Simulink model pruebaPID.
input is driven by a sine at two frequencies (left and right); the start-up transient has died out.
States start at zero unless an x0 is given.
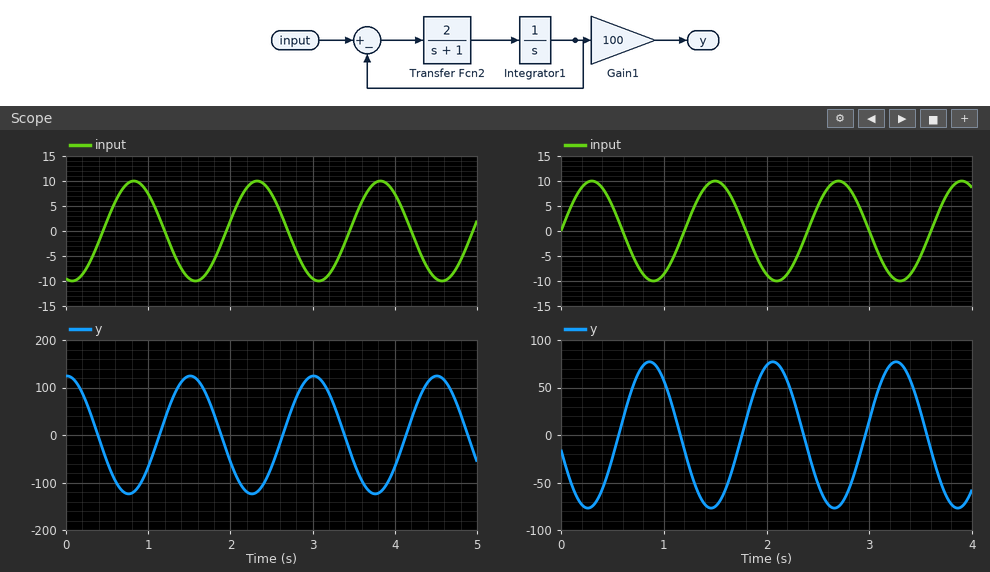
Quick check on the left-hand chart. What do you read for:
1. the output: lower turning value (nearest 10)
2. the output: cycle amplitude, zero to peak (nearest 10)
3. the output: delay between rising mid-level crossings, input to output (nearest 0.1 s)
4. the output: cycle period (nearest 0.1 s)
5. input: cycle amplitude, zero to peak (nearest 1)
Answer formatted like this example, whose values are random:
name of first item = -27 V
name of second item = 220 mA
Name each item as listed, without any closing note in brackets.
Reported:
the output: lower turning value = -120
the output: cycle amplitude, zero to peak = 120
the output: delay between rising mid-level crossings, input to output = 0.7 s
the output: cycle period = 1.5 s
input: cycle amplitude, zero to peak = 10
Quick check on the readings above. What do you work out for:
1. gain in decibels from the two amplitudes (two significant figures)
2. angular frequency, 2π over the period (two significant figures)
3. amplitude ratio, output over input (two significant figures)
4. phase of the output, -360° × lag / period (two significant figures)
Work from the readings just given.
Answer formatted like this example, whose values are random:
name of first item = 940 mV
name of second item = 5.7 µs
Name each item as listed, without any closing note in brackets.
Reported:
gain in decibels from the two amplitudes = 22 dB
angular frequency, 2π over the period = 4.2 rad/s
amplitude ratio, output over input = 12
phase of the output, -360° × lag / period = -170°
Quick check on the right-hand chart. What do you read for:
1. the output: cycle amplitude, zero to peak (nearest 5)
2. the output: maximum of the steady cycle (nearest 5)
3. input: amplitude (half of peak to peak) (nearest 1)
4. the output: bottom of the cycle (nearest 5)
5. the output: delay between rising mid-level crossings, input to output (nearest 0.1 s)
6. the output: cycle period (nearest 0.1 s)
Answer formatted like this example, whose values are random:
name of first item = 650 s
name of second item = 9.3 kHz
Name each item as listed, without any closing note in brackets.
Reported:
the output: cycle amplitude, zero to peak = 75
the output: maximum of the steady cycle = 75
input: amplitude (half of peak to peak) = 10
the output: bottom of the cycle = -75
the output: delay between rising mid-level crossings, input to output = 0.6 s
the output: cycle period = 1.2 s
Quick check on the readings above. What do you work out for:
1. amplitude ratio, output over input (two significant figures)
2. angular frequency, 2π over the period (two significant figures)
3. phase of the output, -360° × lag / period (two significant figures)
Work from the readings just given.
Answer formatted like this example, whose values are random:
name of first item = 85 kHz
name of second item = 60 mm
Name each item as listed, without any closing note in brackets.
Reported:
amplitude ratio, output over input = 7.5
angular frequency, 2π over the period = 5.2 rad/s
phase of the output, -360° × lag / period = -180°
